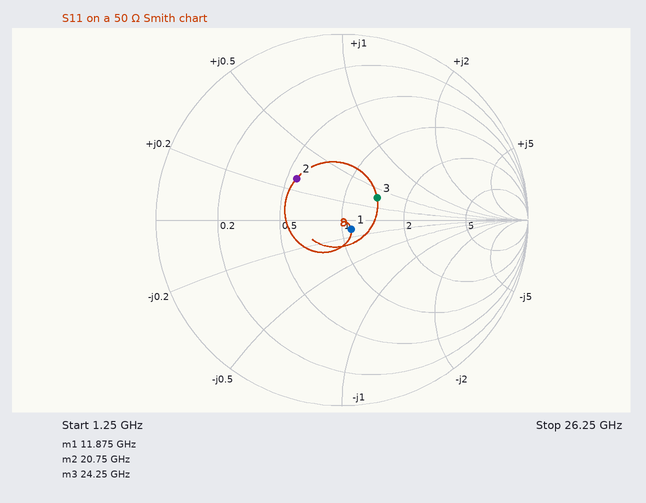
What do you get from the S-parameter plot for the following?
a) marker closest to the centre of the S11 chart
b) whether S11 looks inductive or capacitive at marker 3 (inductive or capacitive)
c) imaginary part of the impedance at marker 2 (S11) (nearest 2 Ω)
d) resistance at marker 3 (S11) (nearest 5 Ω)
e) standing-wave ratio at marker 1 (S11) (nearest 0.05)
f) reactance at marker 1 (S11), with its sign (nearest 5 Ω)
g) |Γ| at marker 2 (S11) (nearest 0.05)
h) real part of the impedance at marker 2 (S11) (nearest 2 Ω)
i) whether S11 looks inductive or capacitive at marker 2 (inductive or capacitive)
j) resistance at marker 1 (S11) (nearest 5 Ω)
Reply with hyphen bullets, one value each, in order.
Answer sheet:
- marker 1
- inductive
- +14 Ω
- 70 Ω
- 1.15
- -5 Ω
- 0.35
- 28 Ω
- inductive
- 55 Ω
